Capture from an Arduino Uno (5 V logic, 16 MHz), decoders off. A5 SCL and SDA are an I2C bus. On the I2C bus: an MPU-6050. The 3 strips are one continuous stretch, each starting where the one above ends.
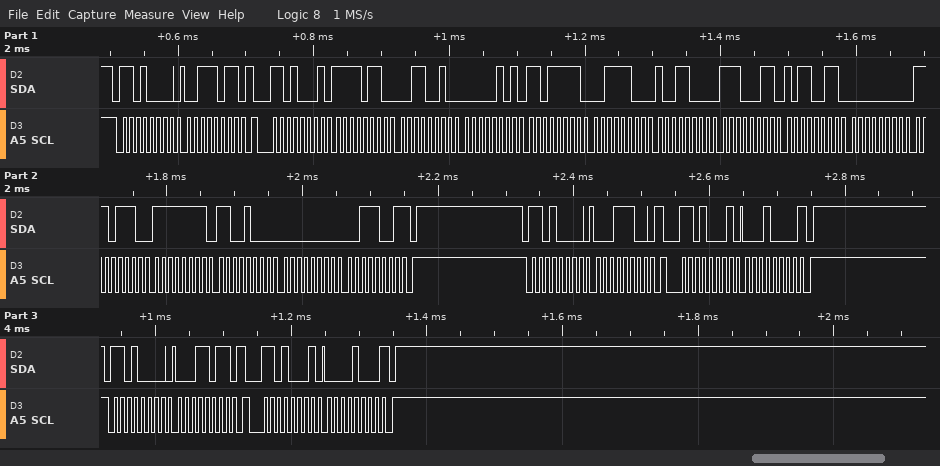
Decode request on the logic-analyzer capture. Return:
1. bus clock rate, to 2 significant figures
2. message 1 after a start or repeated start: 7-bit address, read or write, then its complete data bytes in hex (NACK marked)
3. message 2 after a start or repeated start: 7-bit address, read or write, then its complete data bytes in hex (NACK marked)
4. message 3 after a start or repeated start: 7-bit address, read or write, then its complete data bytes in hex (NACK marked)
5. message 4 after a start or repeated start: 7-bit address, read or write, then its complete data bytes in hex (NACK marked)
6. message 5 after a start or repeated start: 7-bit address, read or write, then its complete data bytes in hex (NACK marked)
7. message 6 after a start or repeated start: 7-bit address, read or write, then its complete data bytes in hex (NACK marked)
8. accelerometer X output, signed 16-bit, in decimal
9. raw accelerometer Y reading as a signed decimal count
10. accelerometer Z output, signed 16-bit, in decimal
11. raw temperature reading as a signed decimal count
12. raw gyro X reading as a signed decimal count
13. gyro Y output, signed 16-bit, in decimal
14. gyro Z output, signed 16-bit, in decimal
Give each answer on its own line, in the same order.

100 kHz
0x68 write: 3B
0x68 read: F6 32 05 DF 3C 98 E3 B3 00 EE FF C8 00 39 NACK
0x68 write: 1C
0x68 read: 10 NACK
0x68 write: 1B
0x68 read: 08 NACK
-2510
1503
15512
-7245
238
-56
57
